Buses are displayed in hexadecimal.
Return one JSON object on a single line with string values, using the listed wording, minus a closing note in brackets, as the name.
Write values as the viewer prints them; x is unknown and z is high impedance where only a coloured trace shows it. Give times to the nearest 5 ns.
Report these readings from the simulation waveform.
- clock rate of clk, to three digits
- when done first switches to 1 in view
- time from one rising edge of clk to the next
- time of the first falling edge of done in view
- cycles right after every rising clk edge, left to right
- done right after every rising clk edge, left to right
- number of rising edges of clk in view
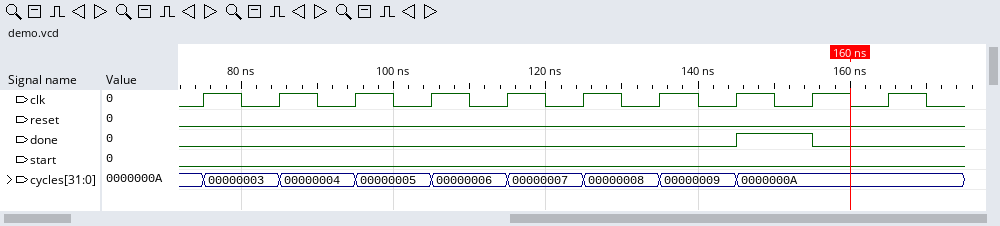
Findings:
{"clock rate of clk, to three digits": "100 MHz", "when done first switches to 1 in view": "145 ns", "time from one rising edge of clk to the next": "10 ns", "time of the first falling edge of done in view": "155 ns", "cycles right after every rising clk edge, left to right": "00000003, 00000004, 00000005, 00000006, 00000007, 00000008, 00000009, 0000000A, 0000000A, 0000000A", "done right after every rising clk edge, left to right": "0 0 0 0 0 0 0 1 0 0", "number of rising edges of clk in view": "10"}
